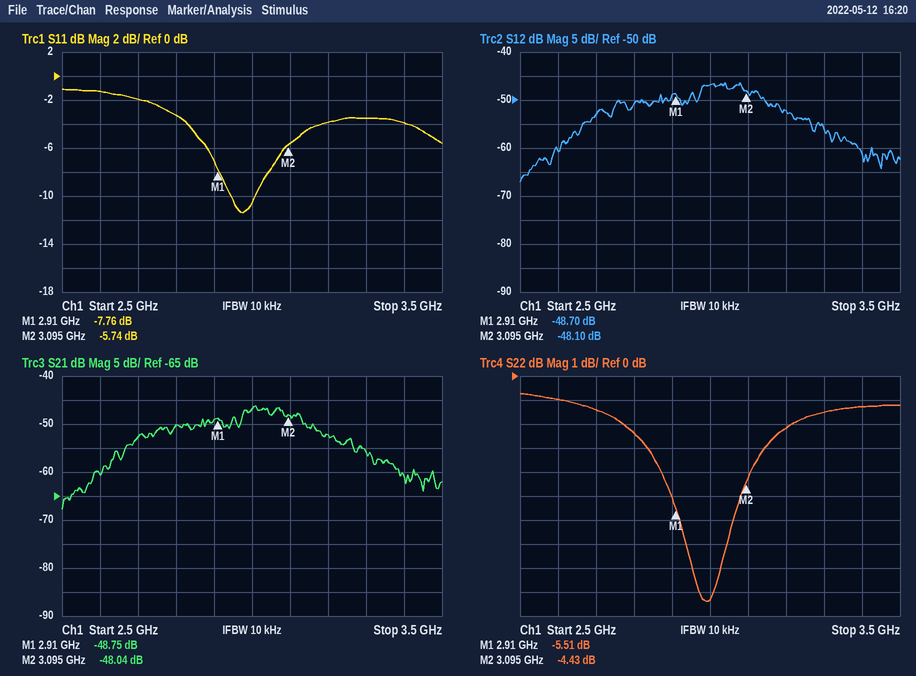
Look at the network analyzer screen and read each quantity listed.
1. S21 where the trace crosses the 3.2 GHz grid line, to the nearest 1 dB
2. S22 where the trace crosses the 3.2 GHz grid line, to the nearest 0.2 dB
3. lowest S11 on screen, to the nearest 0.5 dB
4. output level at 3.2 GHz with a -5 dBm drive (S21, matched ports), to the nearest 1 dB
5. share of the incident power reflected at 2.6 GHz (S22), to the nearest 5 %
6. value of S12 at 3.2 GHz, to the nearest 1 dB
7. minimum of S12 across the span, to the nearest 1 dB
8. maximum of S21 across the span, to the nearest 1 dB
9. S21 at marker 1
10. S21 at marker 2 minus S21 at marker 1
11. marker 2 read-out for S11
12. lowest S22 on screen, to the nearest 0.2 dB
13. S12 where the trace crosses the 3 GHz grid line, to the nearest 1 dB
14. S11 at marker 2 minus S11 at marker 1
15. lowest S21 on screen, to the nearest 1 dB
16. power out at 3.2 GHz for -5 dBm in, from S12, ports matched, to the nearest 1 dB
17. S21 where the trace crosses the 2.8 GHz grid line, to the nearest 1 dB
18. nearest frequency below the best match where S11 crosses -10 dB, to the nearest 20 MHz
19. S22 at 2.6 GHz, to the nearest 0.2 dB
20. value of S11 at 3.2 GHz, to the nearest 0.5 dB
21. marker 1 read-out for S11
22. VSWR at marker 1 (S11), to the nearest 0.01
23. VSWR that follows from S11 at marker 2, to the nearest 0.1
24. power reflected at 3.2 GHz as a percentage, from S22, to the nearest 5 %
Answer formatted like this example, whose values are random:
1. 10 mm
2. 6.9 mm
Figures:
1. -52 dB
2. -2.2 dB
3. -11.5 dB
4. -57 dBm
5. 80 %
6. -52 dB
7. -67 dB
8. -46 dB
9. -48.75 dB
10. 0.71 dB
11. -5.74 dB
12. -9.4 dB
13. -47 dB
14. 2.02 dB
15. -68 dB
16. -57 dBm
17. -50 dB
18. 2.94 GHz
19. -1.0 dB
20. -4.0 dB
21. -7.76 dB
22. 2.39
23. 3.1
24. 60 %
